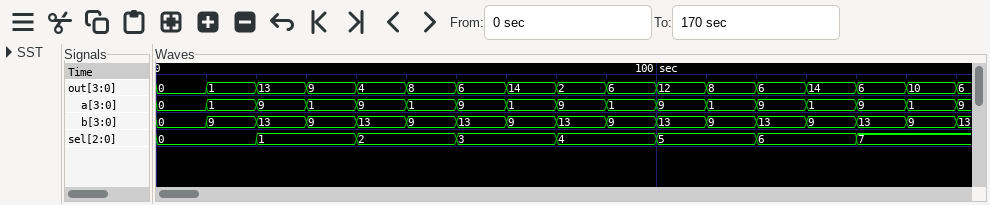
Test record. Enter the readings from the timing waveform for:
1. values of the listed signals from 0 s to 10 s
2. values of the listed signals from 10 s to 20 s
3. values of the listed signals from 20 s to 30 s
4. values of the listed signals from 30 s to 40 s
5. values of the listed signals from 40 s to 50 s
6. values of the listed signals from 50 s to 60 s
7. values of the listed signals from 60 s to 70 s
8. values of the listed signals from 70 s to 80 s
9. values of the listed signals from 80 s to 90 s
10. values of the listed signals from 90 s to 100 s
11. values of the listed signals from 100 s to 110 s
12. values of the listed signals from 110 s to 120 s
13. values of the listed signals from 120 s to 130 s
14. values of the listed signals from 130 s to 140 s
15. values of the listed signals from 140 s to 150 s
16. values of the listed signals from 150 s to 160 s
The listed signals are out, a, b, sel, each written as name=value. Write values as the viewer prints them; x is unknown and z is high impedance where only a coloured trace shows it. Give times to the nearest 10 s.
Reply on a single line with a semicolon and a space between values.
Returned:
out=0, a=0, b=0, sel=0; out=1, a=1, b=9, sel=0; out=13, a=9, b=13, sel=1; out=9, a=1, b=9, sel=1; out=4, a=9, b=13, sel=2; out=8, a=1, b=9, sel=2; out=6, a=9, b=13, sel=3; out=14, a=1, b=9, sel=3; out=2, a=9, b=13, sel=4; out=6, a=1, b=9, sel=4; out=12, a=9, b=13, sel=5; out=8, a=1, b=9, sel=5; out=6, a=9, b=13, sel=6; out=14, a=1, b=9, sel=6; out=6, a=9, b=13, sel=7; out=10, a=1, b=9, sel=7
